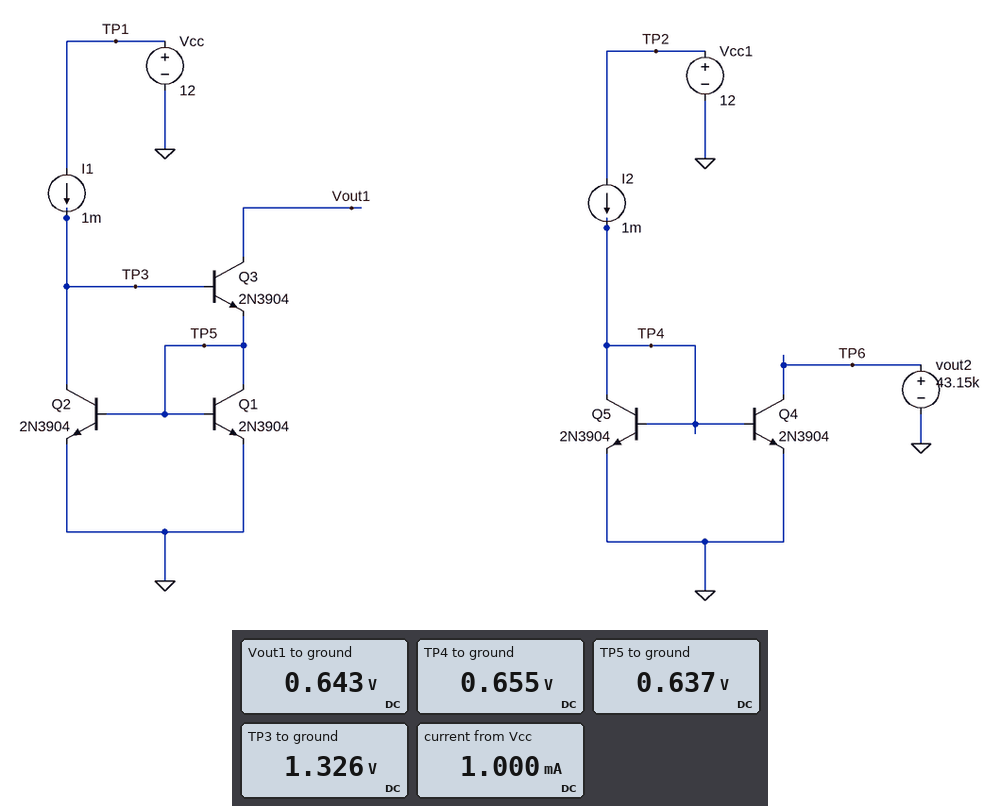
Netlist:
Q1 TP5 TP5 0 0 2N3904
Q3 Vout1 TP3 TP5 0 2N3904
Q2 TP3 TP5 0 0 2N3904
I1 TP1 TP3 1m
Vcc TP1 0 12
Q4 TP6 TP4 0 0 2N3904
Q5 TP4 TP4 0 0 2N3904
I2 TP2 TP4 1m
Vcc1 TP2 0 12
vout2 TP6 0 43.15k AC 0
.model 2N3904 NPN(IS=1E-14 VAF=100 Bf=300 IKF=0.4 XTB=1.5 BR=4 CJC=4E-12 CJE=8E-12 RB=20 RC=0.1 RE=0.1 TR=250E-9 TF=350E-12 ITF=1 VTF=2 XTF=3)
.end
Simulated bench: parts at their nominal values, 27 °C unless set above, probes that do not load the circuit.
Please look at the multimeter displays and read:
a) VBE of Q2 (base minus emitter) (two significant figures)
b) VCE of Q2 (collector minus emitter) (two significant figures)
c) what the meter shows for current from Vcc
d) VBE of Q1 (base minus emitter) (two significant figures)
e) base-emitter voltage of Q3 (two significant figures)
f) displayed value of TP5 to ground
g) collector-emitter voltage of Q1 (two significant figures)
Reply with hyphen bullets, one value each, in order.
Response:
- 640 mV
- 1.3 V
- 1.000 mA
- 640 mV
- 690 mV
- 0.637 V
- 640 mV
